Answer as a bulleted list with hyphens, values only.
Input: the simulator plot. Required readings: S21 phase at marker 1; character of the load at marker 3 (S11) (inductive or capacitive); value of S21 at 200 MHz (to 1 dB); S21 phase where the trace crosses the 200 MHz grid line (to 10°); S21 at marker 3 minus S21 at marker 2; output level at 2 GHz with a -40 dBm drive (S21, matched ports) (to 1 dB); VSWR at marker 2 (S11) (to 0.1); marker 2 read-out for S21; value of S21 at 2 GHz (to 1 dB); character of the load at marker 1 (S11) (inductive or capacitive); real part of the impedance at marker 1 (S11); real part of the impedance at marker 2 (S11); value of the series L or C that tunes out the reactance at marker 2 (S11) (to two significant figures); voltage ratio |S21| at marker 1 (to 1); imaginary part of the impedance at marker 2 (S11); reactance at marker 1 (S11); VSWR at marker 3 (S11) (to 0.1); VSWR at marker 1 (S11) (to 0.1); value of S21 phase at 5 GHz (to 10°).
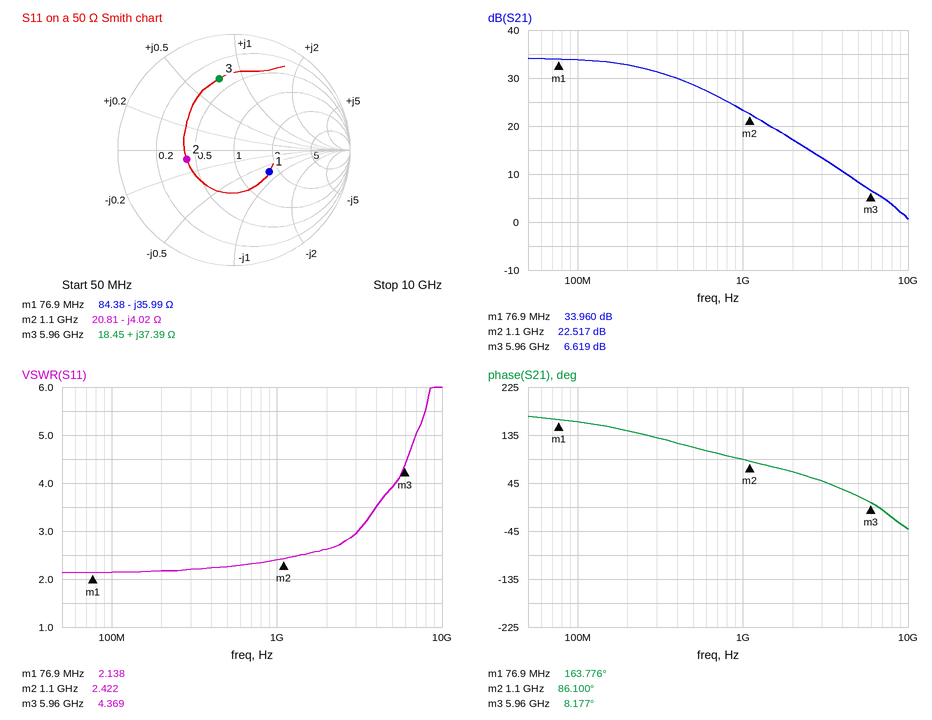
- 163.776°
- inductive
- 33 dB
- 140°
- -15.898 dB
- -23 dBm
- 2.4
- 22.517 dB
- 17 dB
- capacitive
- 84.38 Ω
- 20.81 Ω
- 580 pH
- 50
- -4.02 Ω
- -35.99 Ω
- 4.4
- 2.1
- 20°
